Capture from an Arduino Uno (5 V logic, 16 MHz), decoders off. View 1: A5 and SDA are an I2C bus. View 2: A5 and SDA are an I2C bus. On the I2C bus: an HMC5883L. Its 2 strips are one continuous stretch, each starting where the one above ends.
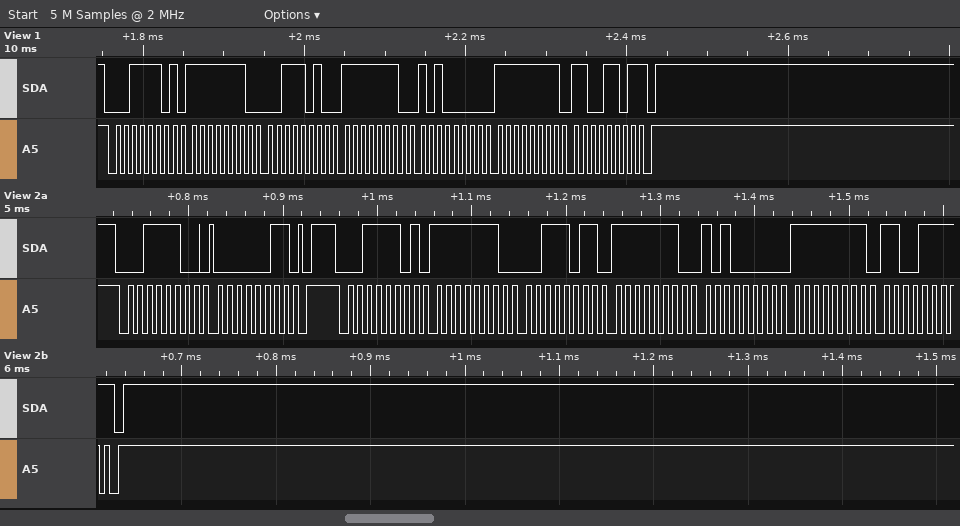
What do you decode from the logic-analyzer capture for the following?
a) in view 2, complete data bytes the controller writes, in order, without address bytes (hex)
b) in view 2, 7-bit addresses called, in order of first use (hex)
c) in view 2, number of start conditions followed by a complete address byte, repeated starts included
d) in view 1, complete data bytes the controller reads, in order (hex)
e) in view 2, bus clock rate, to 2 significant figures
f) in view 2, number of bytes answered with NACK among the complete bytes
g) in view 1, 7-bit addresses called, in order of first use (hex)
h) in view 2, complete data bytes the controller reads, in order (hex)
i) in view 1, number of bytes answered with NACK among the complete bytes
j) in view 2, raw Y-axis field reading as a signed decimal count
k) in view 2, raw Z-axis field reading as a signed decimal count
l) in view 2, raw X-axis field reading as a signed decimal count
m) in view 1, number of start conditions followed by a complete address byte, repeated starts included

03
0x1E
2
FE 3A FE A0 FF CD
100 kHz
1
0x1E
FE 3B FE A0 FF CF
1
-49
-352
-453
1
